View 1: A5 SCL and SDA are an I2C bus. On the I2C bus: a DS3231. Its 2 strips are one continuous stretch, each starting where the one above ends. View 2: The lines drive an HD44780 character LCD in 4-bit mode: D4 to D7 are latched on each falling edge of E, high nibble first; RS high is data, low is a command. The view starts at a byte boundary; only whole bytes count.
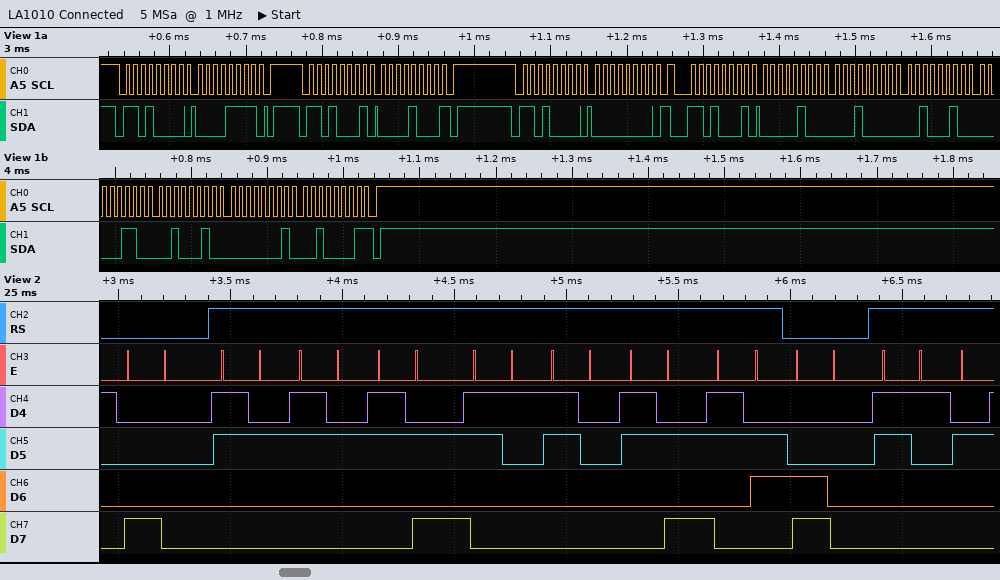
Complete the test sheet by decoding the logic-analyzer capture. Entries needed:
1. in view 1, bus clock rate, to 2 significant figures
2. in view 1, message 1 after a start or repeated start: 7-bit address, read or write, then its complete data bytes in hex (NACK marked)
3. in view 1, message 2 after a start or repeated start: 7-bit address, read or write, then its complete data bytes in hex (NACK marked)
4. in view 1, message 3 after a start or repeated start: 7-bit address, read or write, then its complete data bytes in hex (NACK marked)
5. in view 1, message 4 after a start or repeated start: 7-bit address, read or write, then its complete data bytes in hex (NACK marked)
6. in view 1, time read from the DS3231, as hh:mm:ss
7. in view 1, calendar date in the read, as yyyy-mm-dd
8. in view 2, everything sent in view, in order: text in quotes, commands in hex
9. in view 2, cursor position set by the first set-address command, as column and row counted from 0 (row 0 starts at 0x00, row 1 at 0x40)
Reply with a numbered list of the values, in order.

1. 100 kHz
2. 0x68 write: 0F
3. 0x68 read: 08 NACK
4. 0x68 write: 00
5. 0x68 read: 04 10 22 06 22 01 21 NACK
6. 22:10:04
7. 2021-01-22
8. 0x80 "22:10:6" 0xC0 "1"
9. column 0, row 0
